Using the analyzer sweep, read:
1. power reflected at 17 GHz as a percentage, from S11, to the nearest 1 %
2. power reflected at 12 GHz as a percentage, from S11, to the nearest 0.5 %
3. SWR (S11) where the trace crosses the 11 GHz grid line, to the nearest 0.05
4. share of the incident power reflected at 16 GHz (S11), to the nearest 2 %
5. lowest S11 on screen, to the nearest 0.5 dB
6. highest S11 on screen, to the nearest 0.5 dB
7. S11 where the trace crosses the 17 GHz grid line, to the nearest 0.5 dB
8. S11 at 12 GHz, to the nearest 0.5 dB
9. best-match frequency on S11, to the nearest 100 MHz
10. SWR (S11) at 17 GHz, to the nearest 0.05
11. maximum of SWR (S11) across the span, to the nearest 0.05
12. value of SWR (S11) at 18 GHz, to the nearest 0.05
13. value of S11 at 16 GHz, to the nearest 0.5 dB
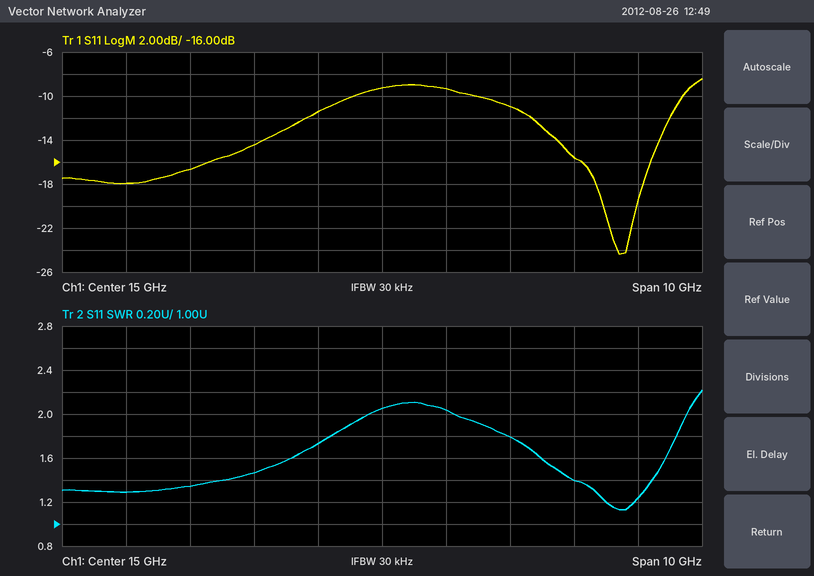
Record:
8 %
2.0 %
1.30
12 %
-24.5 dB
-8.5 dB
-11.0 dB
-16.5 dB
18.7 GHz
1.80
2.20
1.40
-9.5 dB
